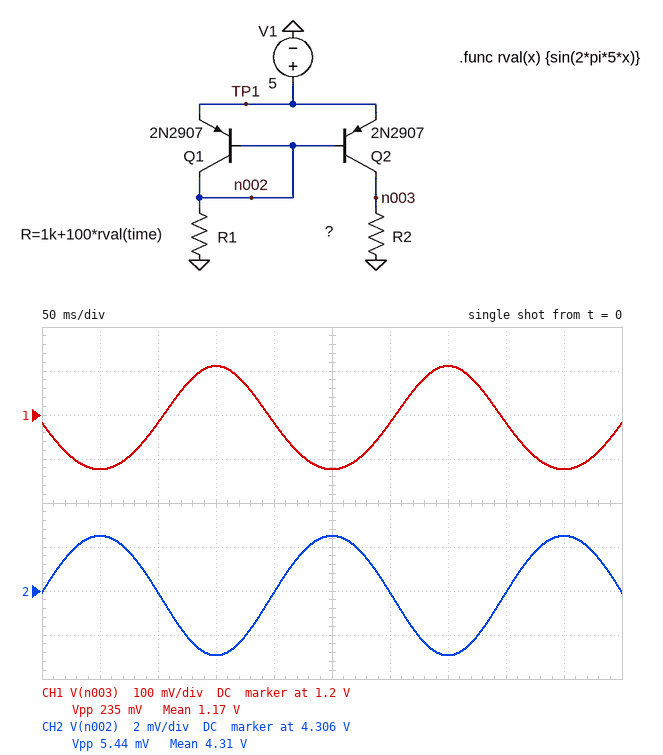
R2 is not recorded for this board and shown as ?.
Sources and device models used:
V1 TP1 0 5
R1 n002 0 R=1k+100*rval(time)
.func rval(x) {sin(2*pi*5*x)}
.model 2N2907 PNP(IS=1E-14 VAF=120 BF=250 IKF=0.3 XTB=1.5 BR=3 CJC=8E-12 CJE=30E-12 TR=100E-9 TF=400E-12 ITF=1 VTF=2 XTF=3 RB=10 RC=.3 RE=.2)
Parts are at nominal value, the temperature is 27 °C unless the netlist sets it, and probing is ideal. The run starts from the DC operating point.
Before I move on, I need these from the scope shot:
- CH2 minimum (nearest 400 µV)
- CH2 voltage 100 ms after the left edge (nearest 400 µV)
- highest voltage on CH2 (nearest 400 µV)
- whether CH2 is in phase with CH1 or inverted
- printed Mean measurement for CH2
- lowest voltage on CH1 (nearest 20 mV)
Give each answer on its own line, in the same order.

4.3032 V
4.3060 V
4.3084 V
inverted
4.31 V
1.08 V
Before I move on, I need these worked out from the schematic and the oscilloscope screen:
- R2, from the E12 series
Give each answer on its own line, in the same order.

270 Ω
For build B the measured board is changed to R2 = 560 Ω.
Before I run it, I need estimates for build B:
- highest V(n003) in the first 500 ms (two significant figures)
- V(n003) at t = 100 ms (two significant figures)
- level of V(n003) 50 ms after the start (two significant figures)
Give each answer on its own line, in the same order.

2.7 V
2.4 V
2.2 V
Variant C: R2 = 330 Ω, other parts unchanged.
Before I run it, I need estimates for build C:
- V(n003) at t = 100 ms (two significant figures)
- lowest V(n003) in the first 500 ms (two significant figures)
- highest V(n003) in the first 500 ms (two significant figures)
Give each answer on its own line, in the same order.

1.4 V
1.3 V
1.6 V
